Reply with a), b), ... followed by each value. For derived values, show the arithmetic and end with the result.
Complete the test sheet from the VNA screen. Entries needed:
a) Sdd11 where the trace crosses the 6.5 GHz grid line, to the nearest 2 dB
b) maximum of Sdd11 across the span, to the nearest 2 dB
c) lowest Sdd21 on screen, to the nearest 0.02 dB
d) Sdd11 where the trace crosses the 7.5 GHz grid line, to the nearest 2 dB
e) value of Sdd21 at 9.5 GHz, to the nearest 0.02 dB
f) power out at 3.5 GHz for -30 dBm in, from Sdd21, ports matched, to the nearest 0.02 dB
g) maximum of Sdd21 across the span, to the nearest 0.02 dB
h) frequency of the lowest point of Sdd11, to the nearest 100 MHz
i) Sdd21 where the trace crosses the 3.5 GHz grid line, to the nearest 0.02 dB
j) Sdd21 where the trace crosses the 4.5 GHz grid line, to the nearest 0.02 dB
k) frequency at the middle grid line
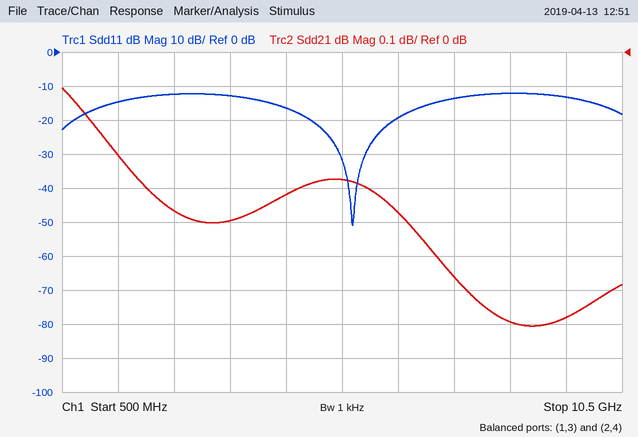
a) -20 dB
b) -12 dB
c) -0.80 dB
d) -14 dB
e) -0.78 dB
f) -30 dBm + (-0.50 dB) = -30.50 dBm
g) -0.10 dB
h) 5.7 GHz
i) -0.50 dB
j) -0.42 dB
k) 5.5 GHz
